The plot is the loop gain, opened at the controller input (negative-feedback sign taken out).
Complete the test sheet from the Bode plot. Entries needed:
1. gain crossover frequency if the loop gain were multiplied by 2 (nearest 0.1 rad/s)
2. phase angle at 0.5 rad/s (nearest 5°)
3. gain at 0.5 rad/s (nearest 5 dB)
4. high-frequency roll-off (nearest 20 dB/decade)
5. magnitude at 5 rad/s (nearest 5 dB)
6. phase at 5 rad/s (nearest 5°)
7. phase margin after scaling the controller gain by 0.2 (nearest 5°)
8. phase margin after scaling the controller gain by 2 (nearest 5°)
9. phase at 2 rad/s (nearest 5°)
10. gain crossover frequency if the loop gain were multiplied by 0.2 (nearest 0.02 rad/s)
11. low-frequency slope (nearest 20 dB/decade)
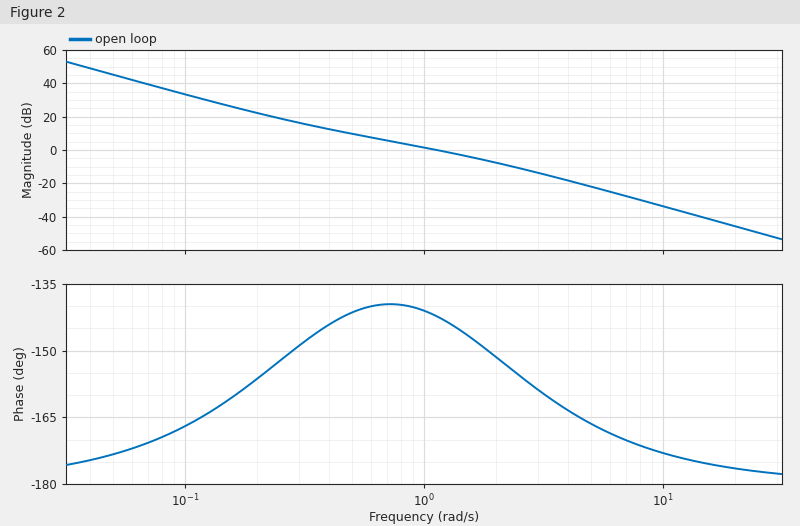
1.8 rad/s
-140°
10 dB
-40 dB/decade
-20 dB
-165°
35°
30°
-150°
0.36 rad/s
-40 dB/decade
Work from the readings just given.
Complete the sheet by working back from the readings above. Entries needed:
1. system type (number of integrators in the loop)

2
